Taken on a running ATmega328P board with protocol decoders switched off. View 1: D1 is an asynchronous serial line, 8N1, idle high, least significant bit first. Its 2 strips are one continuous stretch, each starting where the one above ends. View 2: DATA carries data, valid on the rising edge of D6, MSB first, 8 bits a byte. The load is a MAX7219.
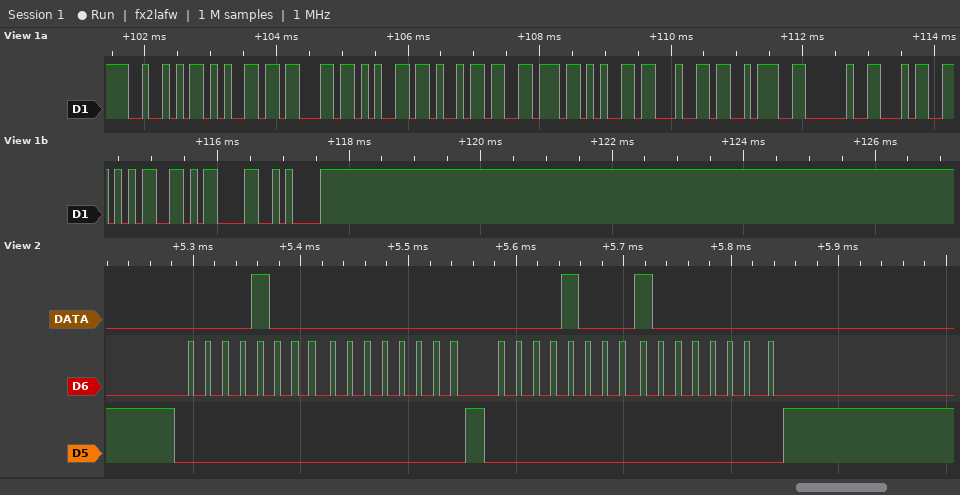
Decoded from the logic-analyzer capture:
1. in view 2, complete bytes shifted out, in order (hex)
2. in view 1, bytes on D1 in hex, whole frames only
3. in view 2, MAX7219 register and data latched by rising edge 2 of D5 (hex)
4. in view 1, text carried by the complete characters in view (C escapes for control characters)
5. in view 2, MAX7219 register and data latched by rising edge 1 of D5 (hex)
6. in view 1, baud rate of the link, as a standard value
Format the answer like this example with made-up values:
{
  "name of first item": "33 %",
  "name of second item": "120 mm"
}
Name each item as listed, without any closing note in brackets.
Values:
{
  "in view 2, complete bytes shifted out, in order": "0x08 0x00 0x08 0x80",
  "in view 1, bytes on D1 in hex, whole frames only": "0x52 0x65 0x63 0x65 0x69 0x76 0x65 0x64 0x3A 0x20 0x34 0x35 0x0D 0x0A",
  "in view 2, MAX7219 register and data latched by rising edge 2 of D5": "register 0x8, data 0x80",
  "in view 1, text carried by the complete characters in view": "\"Received: 45\\r\\n\"",
  "in view 2, MAX7219 register and data latched by rising edge 1 of D5": "register 0x8, data 0x00",
  "in view 1, baud rate of the link, as a standard value": "9600 baud"
}
